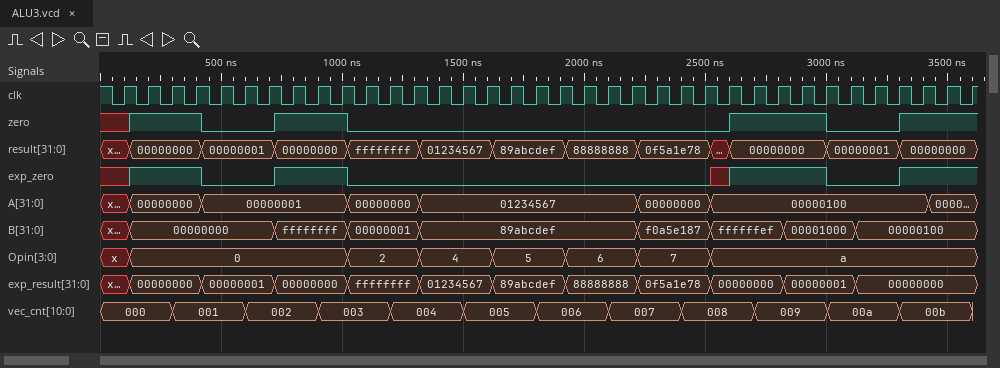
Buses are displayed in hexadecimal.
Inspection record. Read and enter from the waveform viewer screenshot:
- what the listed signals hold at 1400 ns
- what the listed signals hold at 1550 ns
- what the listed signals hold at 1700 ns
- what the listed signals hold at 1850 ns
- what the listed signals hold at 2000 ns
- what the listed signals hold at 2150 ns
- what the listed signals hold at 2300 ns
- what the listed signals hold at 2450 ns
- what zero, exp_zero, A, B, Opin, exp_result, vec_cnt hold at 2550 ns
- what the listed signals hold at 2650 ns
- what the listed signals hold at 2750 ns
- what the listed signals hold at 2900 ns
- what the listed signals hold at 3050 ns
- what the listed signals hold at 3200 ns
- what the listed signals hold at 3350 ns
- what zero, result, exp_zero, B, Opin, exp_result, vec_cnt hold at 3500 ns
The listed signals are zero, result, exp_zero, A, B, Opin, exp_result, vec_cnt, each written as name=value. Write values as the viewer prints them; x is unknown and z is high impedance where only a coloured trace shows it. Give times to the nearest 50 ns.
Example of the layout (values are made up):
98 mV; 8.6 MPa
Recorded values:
zero=0, result=01234567, exp_zero=0, A=01234567, B=89abcdef, Opin=4, exp_result=01234567, vec_cnt=004; zero=0, result=01234567, exp_zero=0, A=01234567, B=89abcdef, Opin=4, exp_result=01234567, vec_cnt=005; zero=0, result=89abcdef, exp_zero=0, A=01234567, B=89abcdef, Opin=5, exp_result=89abcdef, vec_cnt=005; zero=0, result=89abcdef, exp_zero=0, A=01234567, B=89abcdef, Opin=5, exp_result=89abcdef, vec_cnt=006; zero=0, result=88888888, exp_zero=0, A=01234567, B=89abcdef, Opin=6, exp_result=88888888, vec_cnt=006; zero=0, result=88888888, exp_zero=0, A=01234567, B=89abcdef, Opin=6, exp_result=88888888, vec_cnt=007; zero=0, result=0f5a1e78, exp_zero=0, A=00000000, B=f0a5e187, Opin=7, exp_result=0f5a1e78, vec_cnt=007; zero=0, result=0f5a1e78, exp_zero=0, A=00000000, B=f0a5e187, Opin=7, exp_result=0f5a1e78, vec_cnt=008; zero=0, exp_zero=x, A=00000100, B=ffffffef, Opin=a, exp_result=00000000, vec_cnt=008; zero=1, result=00000000, exp_zero=1, A=00000100, B=ffffffef, Opin=a, exp_result=00000000, vec_cnt=008; zero=1, result=00000000, exp_zero=1, A=00000100, B=ffffffef, Opin=a, exp_result=00000000, vec_cnt=009; zero=1, result=00000000, exp_zero=1, A=00000100, B=00001000, Opin=a, exp_result=00000001, vec_cnt=009; zero=0, result=00000001, exp_zero=0, A=00000100, B=00001000, Opin=a, exp_result=00000001, vec_cnt=00a; zero=0, result=00000001, exp_zero=0, A=00000100, B=00000100, Opin=a, exp_result=00000000, vec_cnt=00a; zero=1, result=00000000, exp_zero=1, A=00000100, B=00000100, Opin=a, exp_result=00000000, vec_cnt=00b; zero=1, result=00000000, exp_zero=1, B=00000100, Opin=a, exp_result=00000000, vec_cnt=00b
